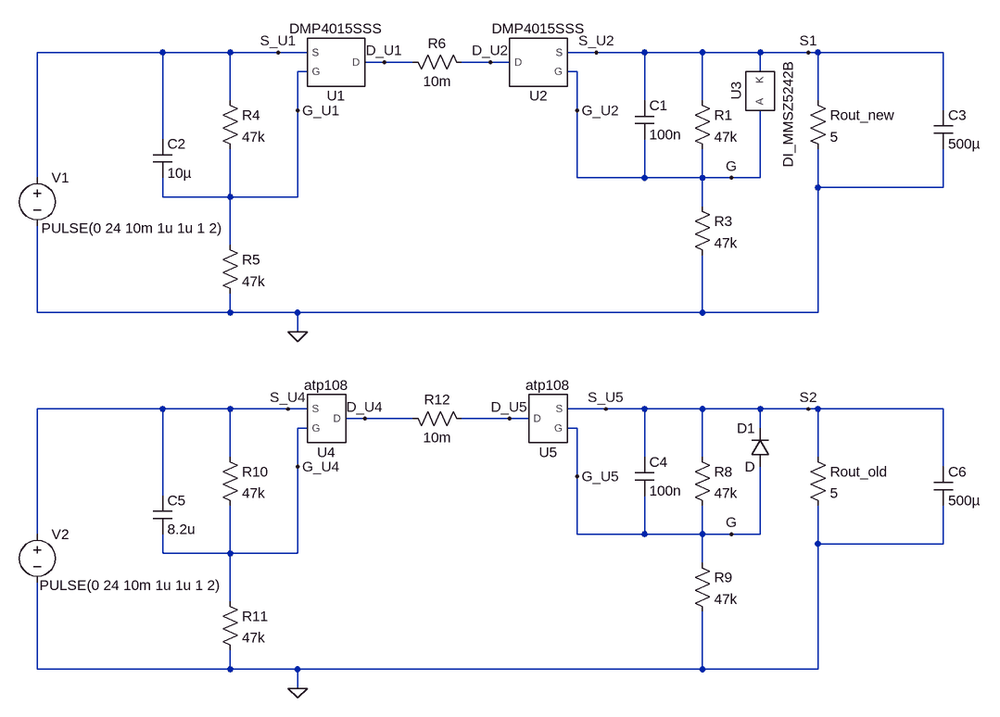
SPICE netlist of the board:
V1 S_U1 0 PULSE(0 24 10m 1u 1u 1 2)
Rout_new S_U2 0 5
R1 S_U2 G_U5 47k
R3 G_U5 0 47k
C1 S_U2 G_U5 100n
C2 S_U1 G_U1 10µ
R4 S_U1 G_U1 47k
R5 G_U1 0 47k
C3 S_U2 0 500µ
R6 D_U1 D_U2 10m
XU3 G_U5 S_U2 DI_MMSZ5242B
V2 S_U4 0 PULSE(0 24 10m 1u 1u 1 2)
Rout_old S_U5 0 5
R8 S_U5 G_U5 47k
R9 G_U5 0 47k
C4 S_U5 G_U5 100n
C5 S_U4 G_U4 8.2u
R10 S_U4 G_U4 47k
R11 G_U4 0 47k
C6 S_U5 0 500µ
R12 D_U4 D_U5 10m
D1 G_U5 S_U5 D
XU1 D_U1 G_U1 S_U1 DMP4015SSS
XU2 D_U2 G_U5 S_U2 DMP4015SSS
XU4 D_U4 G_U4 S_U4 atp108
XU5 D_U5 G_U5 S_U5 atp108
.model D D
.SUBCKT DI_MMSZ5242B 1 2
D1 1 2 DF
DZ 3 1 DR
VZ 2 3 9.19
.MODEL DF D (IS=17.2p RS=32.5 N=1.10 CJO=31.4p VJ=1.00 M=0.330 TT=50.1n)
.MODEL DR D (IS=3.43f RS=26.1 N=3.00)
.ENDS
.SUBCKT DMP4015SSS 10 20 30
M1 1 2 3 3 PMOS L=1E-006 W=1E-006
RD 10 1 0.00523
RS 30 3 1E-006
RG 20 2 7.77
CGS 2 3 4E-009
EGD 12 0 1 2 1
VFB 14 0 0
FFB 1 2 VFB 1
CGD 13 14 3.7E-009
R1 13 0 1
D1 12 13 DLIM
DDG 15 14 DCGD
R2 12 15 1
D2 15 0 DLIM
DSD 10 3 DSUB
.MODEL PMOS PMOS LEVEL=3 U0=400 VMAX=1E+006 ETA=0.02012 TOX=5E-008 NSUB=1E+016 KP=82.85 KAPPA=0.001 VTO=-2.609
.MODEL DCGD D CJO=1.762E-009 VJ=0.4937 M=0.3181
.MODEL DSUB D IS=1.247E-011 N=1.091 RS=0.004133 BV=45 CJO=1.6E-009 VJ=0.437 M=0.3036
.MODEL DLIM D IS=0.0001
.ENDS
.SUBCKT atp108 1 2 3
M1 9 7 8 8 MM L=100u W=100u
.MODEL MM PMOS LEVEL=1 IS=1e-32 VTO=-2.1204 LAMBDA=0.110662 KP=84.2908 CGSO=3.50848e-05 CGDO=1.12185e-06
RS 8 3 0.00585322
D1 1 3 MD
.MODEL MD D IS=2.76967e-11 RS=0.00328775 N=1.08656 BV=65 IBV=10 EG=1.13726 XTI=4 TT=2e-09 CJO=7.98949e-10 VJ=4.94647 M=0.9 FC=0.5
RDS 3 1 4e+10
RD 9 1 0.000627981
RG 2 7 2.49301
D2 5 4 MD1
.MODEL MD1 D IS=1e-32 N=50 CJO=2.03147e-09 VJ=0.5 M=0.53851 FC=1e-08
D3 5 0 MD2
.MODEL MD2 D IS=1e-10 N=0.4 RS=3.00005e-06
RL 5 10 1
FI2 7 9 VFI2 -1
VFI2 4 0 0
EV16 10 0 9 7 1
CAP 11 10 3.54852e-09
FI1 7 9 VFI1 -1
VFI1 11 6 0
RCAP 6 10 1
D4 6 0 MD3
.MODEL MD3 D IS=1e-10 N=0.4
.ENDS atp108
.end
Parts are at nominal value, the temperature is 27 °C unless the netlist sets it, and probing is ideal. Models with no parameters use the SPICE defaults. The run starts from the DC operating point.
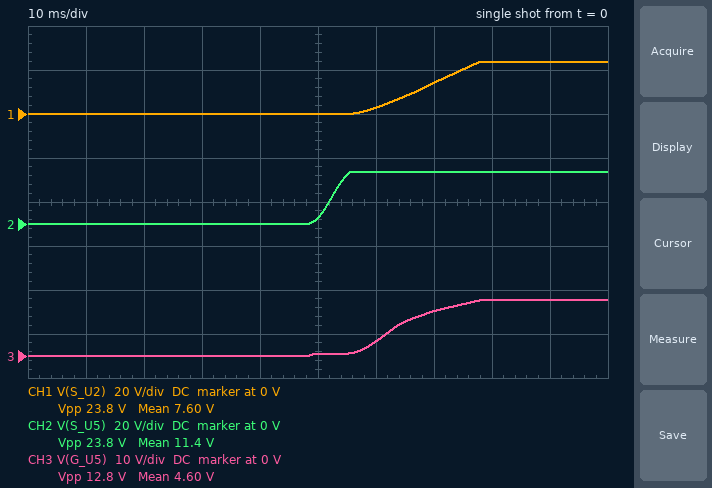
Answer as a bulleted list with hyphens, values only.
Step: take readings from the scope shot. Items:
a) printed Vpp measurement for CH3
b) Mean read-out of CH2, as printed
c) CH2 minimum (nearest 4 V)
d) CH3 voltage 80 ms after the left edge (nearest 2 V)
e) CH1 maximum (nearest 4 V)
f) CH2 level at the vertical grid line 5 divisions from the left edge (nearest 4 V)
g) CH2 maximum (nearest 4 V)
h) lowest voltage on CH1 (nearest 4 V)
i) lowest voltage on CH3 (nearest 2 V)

- 12.8 V
- 11.4 V
- 0 V
- 12 V
- 24 V
- 4 V
- 24 V
- 0 V
- 0 V
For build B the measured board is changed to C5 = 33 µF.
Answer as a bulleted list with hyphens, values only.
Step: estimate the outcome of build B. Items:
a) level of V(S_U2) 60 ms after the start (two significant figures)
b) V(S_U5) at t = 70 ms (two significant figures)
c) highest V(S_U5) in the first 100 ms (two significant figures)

- 2.9 V
- 100 mV
- 1.8 V
